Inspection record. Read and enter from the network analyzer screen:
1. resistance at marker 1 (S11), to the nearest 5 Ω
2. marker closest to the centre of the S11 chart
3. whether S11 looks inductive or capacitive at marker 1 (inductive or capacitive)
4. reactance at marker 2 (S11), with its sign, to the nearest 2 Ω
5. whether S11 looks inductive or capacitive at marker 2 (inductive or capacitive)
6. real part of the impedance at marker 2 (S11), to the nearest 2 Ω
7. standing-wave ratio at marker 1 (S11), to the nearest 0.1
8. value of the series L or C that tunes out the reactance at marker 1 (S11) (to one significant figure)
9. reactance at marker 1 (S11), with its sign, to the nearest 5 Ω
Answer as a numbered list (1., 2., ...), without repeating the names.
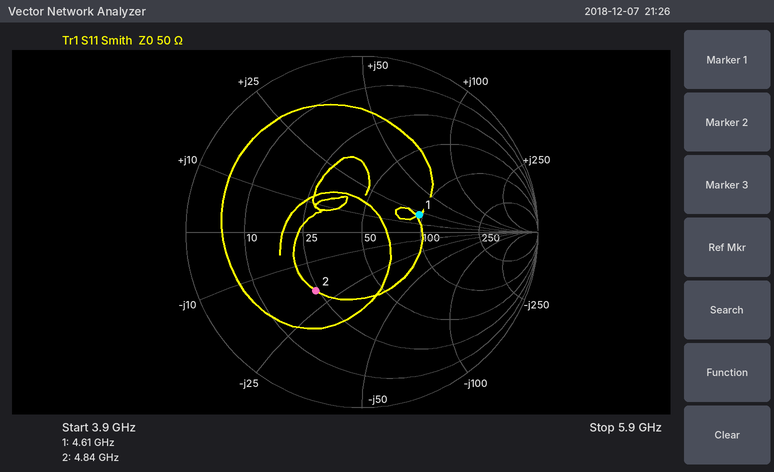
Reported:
1. 95 Ω
2. marker 1
3. inductive
4. -20 Ω
5. capacitive
6. 24 Ω
7. 2.0
8. 2 pF
9. +20 Ω
